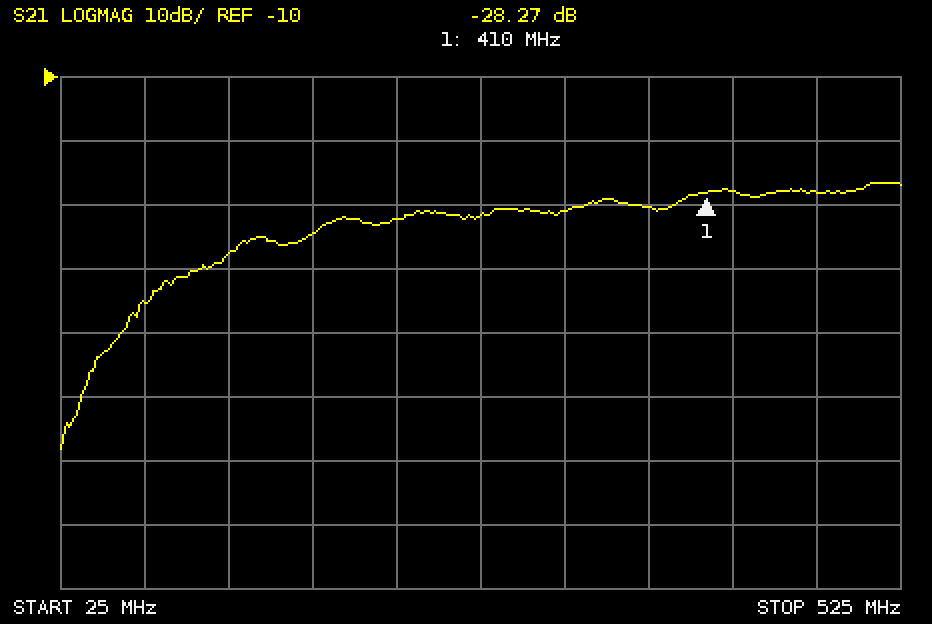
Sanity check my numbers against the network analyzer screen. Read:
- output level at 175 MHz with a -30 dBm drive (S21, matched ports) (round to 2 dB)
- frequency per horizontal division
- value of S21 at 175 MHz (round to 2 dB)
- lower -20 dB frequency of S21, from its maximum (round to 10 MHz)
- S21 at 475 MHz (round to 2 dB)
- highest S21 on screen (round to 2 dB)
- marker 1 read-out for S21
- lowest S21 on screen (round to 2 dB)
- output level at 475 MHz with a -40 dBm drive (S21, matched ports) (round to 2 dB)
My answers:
-64 dBm
50 MHz
-34 dB
70 MHz
-28 dB
-26 dB
-28.27 dB
-68 dB
-68 dBm
